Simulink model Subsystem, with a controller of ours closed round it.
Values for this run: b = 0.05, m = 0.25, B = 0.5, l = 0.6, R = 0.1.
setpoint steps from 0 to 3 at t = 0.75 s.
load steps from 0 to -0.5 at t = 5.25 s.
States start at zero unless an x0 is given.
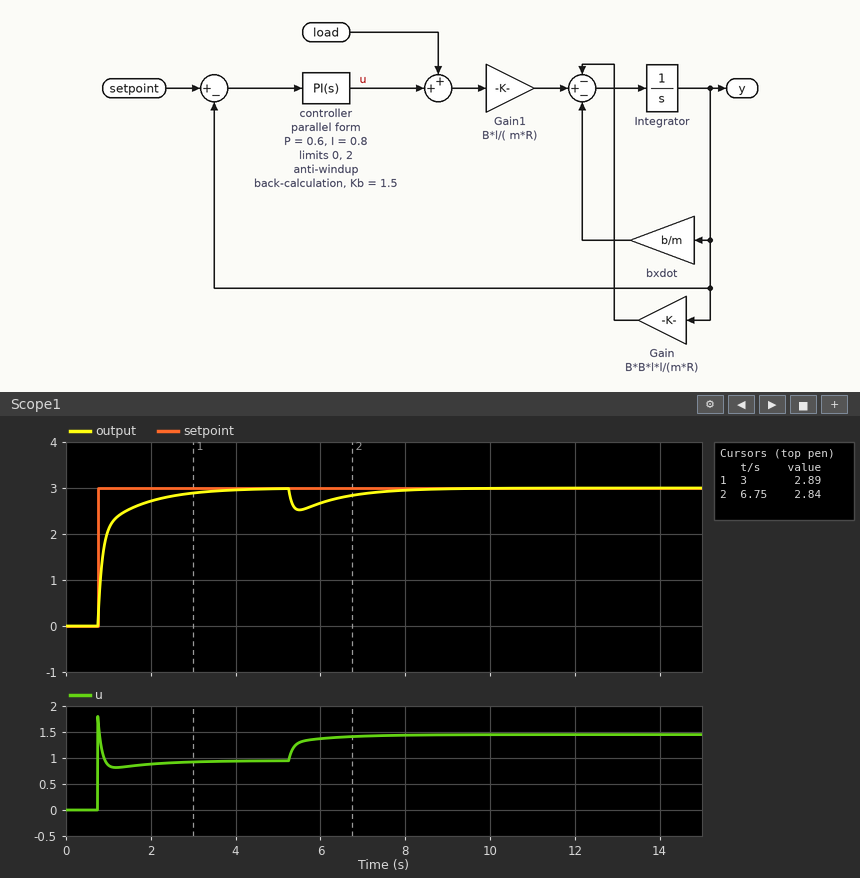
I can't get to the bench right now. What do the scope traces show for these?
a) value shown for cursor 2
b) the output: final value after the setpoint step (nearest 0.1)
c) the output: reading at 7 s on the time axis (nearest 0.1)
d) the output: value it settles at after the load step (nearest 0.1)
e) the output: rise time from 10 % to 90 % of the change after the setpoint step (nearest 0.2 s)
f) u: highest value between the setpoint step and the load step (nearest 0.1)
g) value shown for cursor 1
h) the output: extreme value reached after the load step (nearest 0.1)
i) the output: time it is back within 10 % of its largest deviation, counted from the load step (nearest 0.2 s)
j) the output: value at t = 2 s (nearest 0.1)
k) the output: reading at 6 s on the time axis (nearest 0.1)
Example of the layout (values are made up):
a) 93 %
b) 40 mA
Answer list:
a) 2.84
b) 3.0
c) 2.9
d) 3.0
e) 1.2 s
f) 1.8
g) 2.89
h) 2.5
i) 2.8 s
j) 2.7
k) 2.7
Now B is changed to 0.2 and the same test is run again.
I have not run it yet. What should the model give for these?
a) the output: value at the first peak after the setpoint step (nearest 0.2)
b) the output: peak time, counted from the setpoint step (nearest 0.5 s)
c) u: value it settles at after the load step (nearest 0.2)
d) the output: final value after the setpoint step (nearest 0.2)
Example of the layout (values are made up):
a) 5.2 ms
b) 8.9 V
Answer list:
a) 3.2
b) 1.5 s
c) 1.0
d) 3.0
